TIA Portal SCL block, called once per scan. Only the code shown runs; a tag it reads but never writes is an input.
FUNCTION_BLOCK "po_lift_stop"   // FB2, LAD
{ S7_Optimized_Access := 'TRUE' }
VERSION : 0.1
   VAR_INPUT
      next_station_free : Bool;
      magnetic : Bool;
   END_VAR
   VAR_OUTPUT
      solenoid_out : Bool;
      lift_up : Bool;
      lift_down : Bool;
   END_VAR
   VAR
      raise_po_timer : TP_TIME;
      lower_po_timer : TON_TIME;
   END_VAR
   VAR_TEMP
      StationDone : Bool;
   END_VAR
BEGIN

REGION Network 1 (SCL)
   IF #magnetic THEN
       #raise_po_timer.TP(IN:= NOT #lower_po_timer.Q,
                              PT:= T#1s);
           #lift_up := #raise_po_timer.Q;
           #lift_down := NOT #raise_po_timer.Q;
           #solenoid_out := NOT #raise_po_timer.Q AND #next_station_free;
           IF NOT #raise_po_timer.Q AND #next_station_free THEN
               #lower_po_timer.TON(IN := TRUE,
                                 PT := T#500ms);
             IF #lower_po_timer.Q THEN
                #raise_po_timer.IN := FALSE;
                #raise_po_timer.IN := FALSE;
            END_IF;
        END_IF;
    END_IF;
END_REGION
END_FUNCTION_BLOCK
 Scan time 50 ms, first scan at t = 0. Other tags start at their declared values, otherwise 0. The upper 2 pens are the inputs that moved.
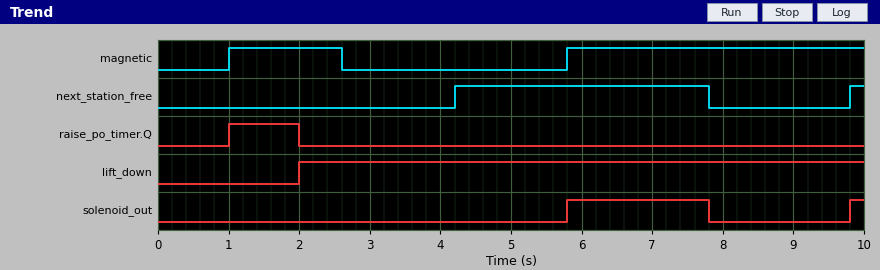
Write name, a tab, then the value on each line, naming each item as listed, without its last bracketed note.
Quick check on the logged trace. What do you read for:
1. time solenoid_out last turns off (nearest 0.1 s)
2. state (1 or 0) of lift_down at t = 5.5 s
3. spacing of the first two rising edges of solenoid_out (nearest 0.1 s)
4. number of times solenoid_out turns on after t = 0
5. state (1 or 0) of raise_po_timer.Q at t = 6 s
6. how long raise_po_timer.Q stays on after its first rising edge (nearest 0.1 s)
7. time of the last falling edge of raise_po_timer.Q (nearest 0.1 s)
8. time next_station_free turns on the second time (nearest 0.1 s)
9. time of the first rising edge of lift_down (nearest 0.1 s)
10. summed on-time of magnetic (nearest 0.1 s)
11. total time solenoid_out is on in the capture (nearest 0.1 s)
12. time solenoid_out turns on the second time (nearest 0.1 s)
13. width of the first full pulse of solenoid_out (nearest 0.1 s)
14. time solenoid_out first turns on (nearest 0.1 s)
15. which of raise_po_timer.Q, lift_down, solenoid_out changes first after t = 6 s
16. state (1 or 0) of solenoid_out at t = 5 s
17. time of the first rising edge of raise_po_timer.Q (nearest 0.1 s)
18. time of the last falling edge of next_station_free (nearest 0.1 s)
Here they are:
time solenoid_out last turns off	7.8 s
state (1 or 0) of lift_down at t = 5.5 s	1
spacing of the first two rising edges of solenoid_out	4.0 s
number of times solenoid_out turns on after t = 0	2
state (1 or 0) of raise_po_timer.Q at t = 6 s	0
how long raise_po_timer.Q stays on after its first rising edge	1.0 s
time of the last falling edge of raise_po_timer.Q	2.0 s
time next_station_free turns on the second time	9.8 s
time of the first rising edge of lift_down	2.0 s
summed on-time of magnetic	5.8 s
total time solenoid_out is on in the capture	2.2 s
time solenoid_out turns on the second time	9.8 s
width of the first full pulse of solenoid_out	2.0 s
time solenoid_out first turns on	5.8 s
which of raise_po_timer.Q, lift_down, solenoid_out changes first after t = 6 s	solenoid_out
state (1 or 0) of solenoid_out at t = 5 s	0
time of the first rising edge of raise_po_timer.Q	1.0 s
time of the last falling edge of next_station_free	7.8 s
